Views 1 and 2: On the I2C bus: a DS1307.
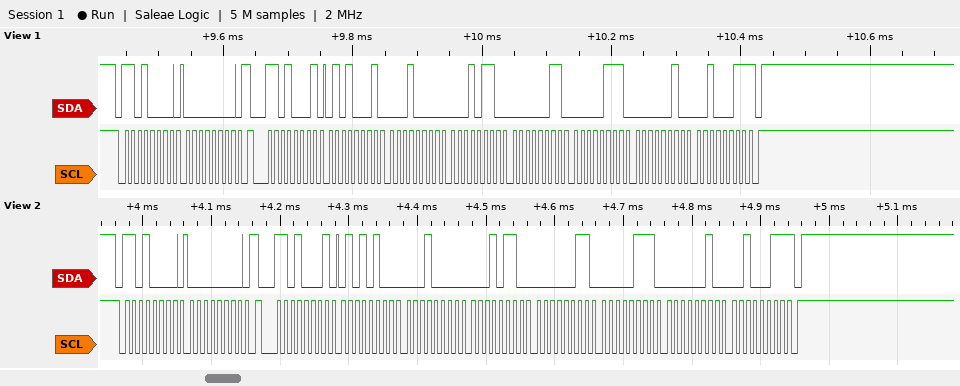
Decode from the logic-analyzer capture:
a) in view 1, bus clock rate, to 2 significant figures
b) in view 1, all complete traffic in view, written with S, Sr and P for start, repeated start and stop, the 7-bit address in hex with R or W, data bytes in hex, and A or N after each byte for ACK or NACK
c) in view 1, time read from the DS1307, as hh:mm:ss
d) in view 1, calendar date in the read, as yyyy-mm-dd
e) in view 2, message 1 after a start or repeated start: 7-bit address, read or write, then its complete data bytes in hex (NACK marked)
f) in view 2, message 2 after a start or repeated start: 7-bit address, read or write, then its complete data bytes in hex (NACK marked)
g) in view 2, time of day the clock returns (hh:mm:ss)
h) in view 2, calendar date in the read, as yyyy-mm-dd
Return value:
100 kHz
S 68W A 00 A Sr 68R A 51 A 10 A 16 A 03 A 07 A 02 A 23 N P
16:10:51
2023-02-07
0x68 write: 00
0x68 read: 54 10 16 03 07 02 23 NACK
16:10:54
2023-02-07
